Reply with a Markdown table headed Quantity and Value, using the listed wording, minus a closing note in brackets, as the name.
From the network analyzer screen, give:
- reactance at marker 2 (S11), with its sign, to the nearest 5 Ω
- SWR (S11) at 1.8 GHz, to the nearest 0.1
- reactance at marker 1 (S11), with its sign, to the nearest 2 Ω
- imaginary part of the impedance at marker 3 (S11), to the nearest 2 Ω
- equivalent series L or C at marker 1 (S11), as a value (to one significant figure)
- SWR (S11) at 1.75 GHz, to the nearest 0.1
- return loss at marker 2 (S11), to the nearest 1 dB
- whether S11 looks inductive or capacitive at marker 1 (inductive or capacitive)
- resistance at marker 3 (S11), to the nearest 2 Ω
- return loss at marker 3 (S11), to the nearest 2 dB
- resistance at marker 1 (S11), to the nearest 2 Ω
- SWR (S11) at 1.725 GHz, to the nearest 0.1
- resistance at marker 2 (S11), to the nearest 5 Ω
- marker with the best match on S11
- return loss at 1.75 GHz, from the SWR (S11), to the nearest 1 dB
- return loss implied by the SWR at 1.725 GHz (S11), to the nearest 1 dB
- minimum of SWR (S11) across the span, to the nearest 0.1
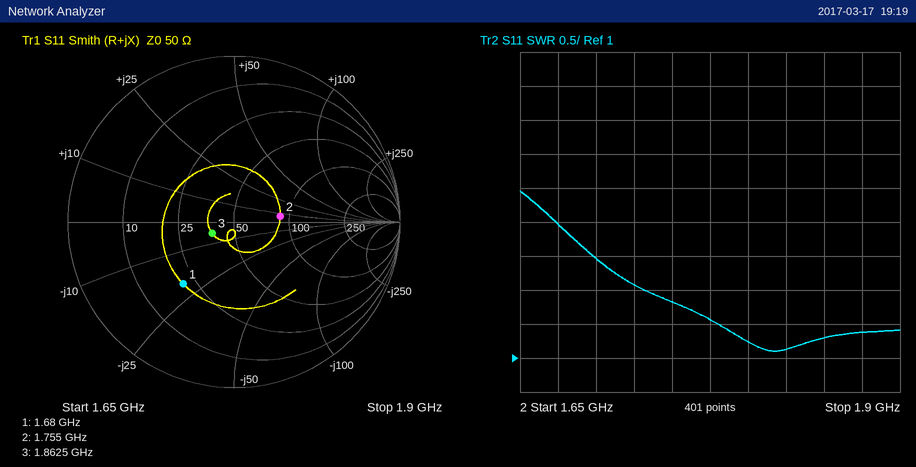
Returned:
| Quantity | Value |
|---|---|
| reactance at marker 2 (S11), with its sign, to the nearest 5 Ω | +5 Ω |
| SWR (S11) at 1.8 GHz, to the nearest 0.1 | 1.2 |
| reactance at marker 1 (S11), with its sign, to the nearest 2 Ω | -20 Ω |
| imaginary part of the impedance at marker 3 (S11), to the nearest 2 Ω | -6 Ω |
| equivalent series L or C at marker 1 (S11), as a value | 5 pF |
| SWR (S11) at 1.75 GHz, to the nearest 0.1 | 1.8 |
| return loss at marker 2 (S11), to the nearest 1 dB | 11 dB |
| whether S11 looks inductive or capacitive at marker 1 | capacitive |
| resistance at marker 3 (S11), to the nearest 2 Ω | 38 Ω |
| return loss at marker 3 (S11), to the nearest 2 dB | 16 dB |
| resistance at marker 1 (S11), to the nearest 2 Ω | 20 Ω |
| SWR (S11) at 1.725 GHz, to the nearest 0.1 | 2.1 |
| resistance at marker 2 (S11), to the nearest 5 Ω | 90 Ω |
| marker with the best match on S11 | marker 3 |
| return loss at 1.75 GHz, from the SWR (S11), to the nearest 1 dB | 11 dB |
| return loss implied by the SWR at 1.725 GHz (S11), to the nearest 1 dB | 9 dB |
| minimum of SWR (S11) across the span, to the nearest 0.1 | 1.1 |
